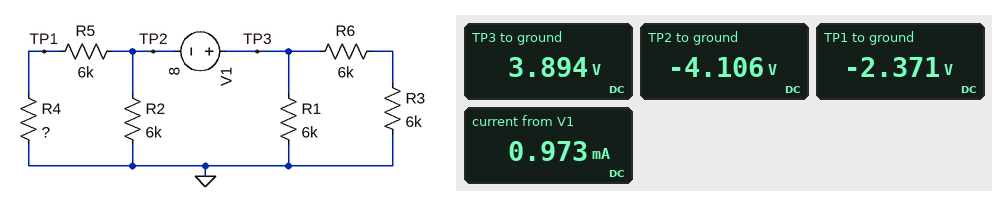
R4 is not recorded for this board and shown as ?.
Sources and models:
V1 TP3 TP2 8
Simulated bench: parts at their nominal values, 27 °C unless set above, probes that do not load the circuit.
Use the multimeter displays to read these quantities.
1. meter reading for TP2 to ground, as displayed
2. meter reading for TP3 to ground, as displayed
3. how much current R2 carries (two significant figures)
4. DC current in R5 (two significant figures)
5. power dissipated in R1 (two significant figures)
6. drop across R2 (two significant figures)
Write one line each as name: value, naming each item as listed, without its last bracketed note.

meter reading for TP2 to ground, as displayed: -4.106 V
meter reading for TP3 to ground, as displayed: 3.894 V
how much current R2 carries: 680 µA
DC current in R5: 290 µA
power dissipated in R1: 2.5 mW
drop across R2: 4.1 V
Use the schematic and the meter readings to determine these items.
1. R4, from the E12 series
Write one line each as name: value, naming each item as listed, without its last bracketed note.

R4, from the E12 series: 8.2 kΩ
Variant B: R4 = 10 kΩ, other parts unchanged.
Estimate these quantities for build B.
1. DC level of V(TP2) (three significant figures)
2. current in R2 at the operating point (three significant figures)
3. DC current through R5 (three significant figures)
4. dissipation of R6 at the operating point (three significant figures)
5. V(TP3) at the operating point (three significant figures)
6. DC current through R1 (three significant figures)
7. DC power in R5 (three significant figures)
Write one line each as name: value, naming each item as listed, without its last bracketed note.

DC level of V(TP2): -4.17 V
current in R2 at the operating point: 696 µA
DC current through R5: 261 µA
dissipation of R6 at the operating point: 610 µW
V(TP3) at the operating point: 3.83 V
DC current through R1: 638 µA
DC power in R5: 408 µW
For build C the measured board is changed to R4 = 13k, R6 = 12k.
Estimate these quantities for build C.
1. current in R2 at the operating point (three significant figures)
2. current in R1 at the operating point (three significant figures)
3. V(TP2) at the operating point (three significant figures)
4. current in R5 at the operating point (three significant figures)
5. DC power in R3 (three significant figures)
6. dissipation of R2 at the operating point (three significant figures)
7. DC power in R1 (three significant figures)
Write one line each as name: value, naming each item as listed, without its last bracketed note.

current in R2 at the operating point: 671 µA
current in R1 at the operating point: 662 µA
V(TP2) at the operating point: -4.03 V
current in R5 at the operating point: 212 µA
DC power in R3: 292 µW
dissipation of R2 at the operating point: 2.70 mW
DC power in R1: 2.63 mW
